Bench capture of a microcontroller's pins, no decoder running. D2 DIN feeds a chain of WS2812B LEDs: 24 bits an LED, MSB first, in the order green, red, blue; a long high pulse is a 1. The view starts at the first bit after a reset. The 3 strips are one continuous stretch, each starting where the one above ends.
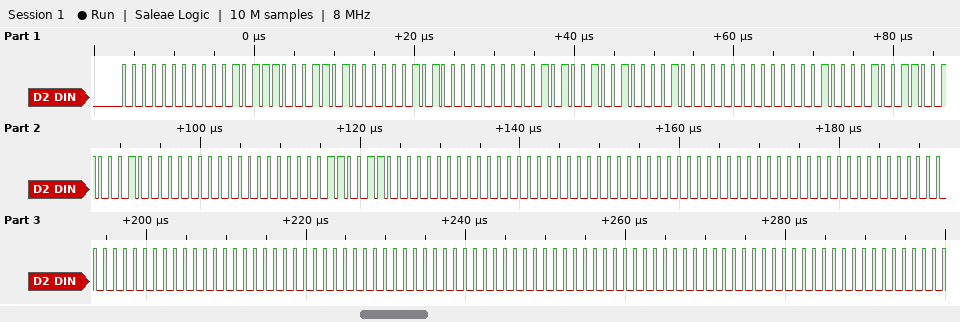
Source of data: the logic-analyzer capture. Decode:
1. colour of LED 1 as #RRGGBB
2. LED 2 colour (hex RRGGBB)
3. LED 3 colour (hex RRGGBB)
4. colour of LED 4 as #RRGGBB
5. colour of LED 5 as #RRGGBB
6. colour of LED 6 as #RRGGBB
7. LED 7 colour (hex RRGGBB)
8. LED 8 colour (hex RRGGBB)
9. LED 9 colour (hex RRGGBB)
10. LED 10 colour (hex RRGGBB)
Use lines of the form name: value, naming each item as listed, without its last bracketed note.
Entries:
colour of LED 1 as #RRGGBB: #17001A
LED 2 colour: #000529
LED 3 colour: #002102
colour of LED 4 as #RRGGBB: #221300
colour of LED 5 as #RRGGBB: #330000
colour of LED 6 as #RRGGBB: #000000
LED 7 colour: #000000
LED 8 colour: #000000
LED 9 colour: #000000
LED 10 colour: #000000
